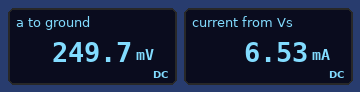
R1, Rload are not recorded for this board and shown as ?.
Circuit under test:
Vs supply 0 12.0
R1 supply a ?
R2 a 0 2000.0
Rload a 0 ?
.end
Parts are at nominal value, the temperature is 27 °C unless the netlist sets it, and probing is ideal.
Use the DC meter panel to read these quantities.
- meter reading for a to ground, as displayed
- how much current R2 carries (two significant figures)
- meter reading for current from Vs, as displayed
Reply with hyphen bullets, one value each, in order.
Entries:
- 249.7 mV
- 120 µA
- 6.53 mA
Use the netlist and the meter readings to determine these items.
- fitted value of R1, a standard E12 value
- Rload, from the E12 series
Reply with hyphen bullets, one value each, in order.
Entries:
- 1.8 kΩ
- 39 Ω
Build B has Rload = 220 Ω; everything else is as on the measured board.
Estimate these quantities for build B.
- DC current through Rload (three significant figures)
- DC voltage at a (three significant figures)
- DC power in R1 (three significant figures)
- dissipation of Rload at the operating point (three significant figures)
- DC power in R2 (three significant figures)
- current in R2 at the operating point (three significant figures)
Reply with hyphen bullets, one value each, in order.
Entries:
- 5.41 mA
- 1.19 V
- 64.9 mW
- 6.44 mW
- 708 µW
- 595 µA
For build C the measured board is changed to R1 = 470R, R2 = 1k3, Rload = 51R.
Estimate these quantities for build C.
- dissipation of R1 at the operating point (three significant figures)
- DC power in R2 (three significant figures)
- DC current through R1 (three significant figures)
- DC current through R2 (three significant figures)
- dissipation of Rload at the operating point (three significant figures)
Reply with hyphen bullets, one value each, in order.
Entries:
- 251 mW
- 990 µW
- 23.1 mA
- 873 µA
- 25.2 mW
